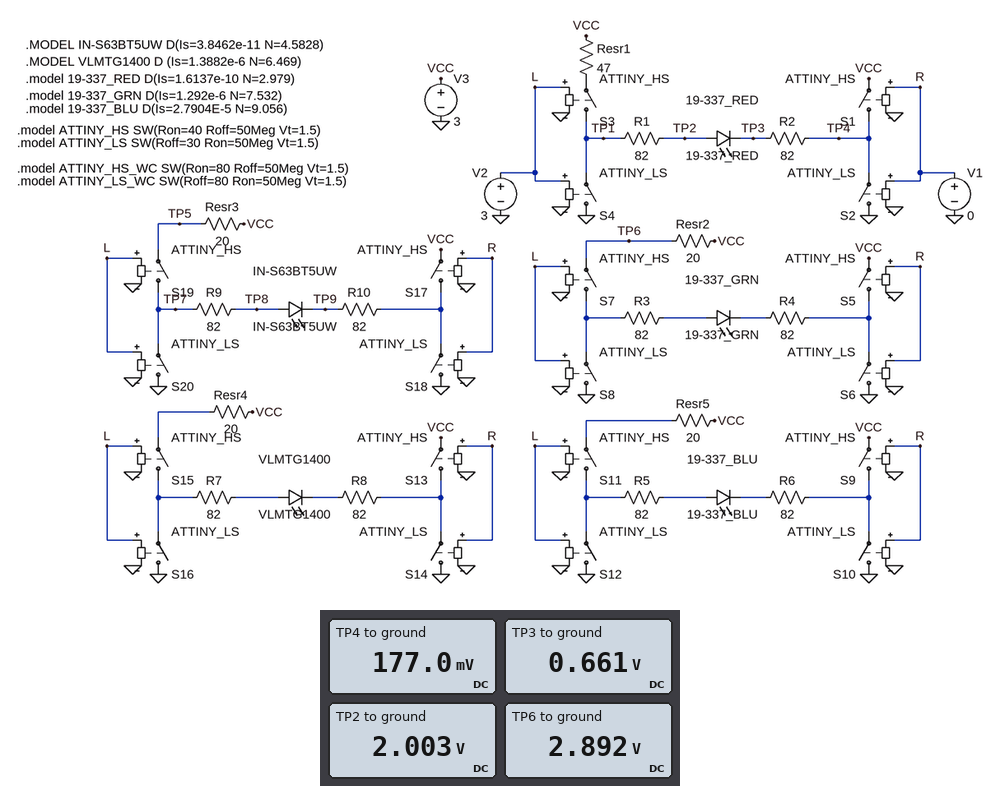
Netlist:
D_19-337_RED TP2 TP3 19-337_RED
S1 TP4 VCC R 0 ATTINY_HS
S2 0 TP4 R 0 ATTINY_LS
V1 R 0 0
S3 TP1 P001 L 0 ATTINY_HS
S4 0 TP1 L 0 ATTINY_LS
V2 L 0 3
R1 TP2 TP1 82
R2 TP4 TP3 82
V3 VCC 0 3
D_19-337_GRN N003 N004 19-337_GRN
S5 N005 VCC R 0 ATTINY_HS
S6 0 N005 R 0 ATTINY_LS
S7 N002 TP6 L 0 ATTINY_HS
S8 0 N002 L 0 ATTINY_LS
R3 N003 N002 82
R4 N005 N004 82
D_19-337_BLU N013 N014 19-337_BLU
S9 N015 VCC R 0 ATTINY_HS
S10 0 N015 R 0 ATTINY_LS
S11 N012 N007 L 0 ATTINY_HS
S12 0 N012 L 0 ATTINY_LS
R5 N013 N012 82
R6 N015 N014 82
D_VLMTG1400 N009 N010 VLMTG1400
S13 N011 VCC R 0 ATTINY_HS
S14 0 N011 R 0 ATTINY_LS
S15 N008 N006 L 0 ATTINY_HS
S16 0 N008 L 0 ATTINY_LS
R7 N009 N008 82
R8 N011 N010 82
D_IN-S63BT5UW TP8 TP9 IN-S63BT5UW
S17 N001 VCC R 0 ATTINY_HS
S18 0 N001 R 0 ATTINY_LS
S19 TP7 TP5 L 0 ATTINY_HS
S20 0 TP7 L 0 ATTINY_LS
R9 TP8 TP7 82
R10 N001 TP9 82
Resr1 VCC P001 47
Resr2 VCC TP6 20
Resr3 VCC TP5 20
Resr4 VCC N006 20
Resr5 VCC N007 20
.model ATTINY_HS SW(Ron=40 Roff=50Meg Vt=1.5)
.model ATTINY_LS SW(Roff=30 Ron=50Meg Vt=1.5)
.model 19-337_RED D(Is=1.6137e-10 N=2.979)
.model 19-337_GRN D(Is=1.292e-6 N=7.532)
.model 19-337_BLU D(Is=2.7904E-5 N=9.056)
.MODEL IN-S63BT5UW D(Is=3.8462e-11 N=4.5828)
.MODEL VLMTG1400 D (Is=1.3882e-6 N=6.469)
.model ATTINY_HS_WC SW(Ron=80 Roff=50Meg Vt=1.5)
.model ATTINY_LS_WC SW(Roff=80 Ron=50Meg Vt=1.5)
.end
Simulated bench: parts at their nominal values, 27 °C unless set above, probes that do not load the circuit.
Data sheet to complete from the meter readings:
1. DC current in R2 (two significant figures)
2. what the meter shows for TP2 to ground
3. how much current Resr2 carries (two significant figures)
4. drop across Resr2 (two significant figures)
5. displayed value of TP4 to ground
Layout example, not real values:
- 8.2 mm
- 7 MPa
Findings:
- 5.9 mA
- 2.003 V
- 5.4 mA
- 110 mV
- 177.0 mV
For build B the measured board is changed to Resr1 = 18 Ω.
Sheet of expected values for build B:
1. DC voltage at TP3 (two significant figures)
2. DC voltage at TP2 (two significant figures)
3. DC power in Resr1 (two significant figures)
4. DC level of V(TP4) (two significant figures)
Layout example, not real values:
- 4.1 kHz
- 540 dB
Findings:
- 730 mV
- 2.1 V
- 770 µW
- 200 mV
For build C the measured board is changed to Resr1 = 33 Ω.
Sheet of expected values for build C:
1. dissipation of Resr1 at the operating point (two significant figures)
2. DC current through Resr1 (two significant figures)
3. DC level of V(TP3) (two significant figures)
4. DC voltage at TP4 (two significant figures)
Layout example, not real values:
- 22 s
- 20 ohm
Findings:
- 1.3 mW
- 6.2 mA
- 690 mV
- 190 mV
